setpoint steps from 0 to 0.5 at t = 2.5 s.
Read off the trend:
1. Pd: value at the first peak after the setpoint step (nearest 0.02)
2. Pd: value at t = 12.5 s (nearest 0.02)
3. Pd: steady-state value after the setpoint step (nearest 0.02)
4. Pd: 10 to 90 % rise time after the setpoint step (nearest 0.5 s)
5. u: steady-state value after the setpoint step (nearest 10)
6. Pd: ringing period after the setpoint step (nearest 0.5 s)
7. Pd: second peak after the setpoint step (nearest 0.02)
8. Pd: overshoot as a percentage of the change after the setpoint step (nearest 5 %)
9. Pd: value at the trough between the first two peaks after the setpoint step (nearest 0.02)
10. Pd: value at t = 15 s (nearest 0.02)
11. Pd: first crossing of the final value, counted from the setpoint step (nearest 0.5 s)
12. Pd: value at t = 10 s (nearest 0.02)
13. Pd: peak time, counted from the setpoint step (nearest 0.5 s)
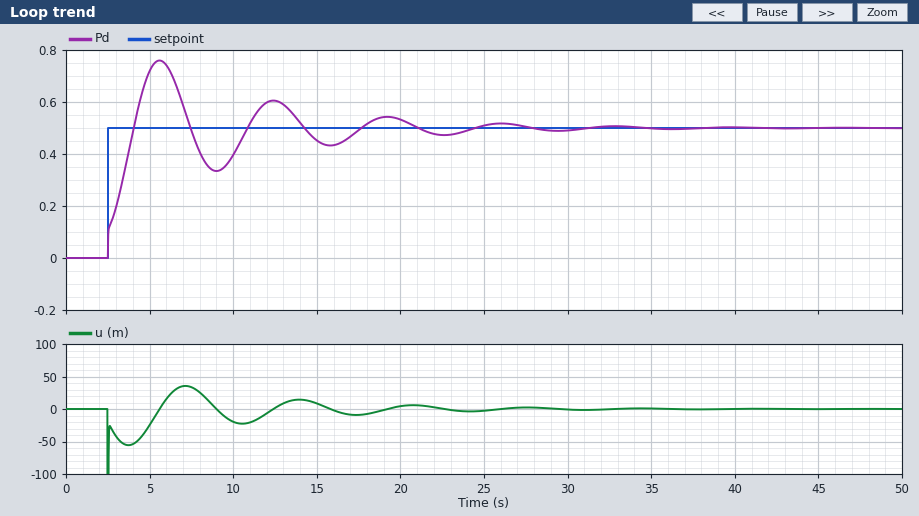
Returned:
0.76
0.60
0.50
1.5 s
0
7.0 s
0.60
50 %
0.34
0.46
1.5 s
0.40
3.0 s
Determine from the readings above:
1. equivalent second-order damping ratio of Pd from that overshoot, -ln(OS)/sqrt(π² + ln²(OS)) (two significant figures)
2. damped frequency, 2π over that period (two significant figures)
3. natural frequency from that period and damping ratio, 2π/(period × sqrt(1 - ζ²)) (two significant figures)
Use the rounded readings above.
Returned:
0.22
0.90 rad/s
0.92 rad/s
